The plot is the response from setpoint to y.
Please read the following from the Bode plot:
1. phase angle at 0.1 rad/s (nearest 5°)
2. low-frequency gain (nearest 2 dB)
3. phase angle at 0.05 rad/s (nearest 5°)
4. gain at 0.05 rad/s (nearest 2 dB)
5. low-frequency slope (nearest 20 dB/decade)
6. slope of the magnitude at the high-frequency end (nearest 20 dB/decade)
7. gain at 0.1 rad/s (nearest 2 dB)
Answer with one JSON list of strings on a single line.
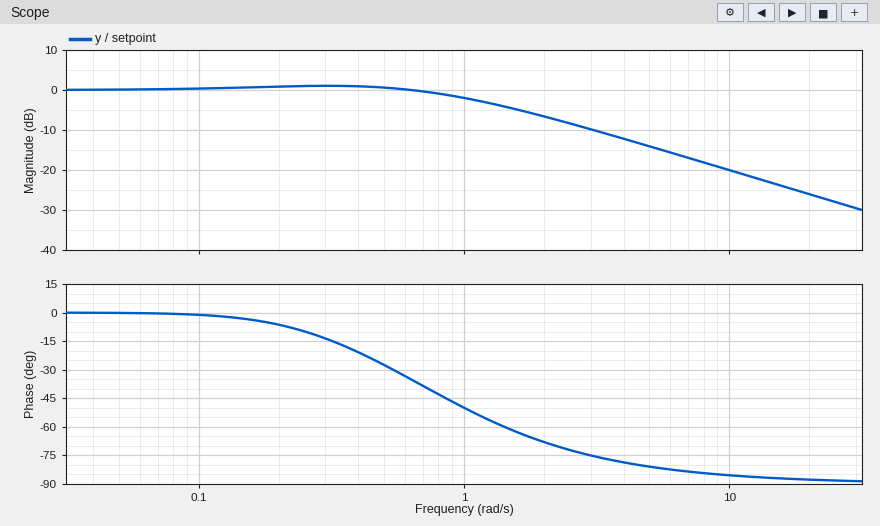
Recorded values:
["0°", "0 dB", "0°", "0 dB", "0 dB/decade", "-20 dB/decade", "0 dB"]
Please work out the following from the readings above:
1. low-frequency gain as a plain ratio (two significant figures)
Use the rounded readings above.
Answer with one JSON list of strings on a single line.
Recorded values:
["1.0"]
